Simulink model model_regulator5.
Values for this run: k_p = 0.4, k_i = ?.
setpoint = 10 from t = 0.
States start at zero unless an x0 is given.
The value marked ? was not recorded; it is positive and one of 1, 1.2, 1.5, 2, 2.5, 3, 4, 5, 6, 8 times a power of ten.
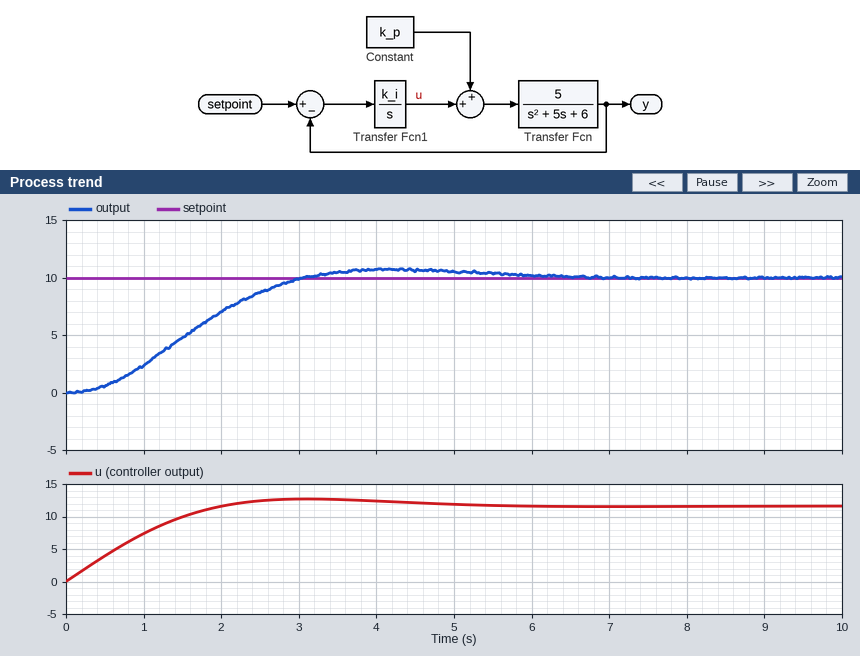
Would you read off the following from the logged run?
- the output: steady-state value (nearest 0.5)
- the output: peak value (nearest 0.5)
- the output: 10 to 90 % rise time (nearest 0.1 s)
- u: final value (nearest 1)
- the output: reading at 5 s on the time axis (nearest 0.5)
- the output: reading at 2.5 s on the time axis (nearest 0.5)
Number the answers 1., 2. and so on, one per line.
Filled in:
1. 10.0
2. 10.5
3. 2.0 s
4. 12
5. 10.5
6. 8.5
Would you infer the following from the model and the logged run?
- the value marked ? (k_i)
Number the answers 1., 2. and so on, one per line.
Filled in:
1. 0.8
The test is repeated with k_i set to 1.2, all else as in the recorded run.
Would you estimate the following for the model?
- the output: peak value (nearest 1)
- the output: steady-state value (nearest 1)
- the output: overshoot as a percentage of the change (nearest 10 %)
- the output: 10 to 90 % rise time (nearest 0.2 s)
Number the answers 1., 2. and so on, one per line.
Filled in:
1. 12
2. 10
3. 20 %
4. 1.4 s
